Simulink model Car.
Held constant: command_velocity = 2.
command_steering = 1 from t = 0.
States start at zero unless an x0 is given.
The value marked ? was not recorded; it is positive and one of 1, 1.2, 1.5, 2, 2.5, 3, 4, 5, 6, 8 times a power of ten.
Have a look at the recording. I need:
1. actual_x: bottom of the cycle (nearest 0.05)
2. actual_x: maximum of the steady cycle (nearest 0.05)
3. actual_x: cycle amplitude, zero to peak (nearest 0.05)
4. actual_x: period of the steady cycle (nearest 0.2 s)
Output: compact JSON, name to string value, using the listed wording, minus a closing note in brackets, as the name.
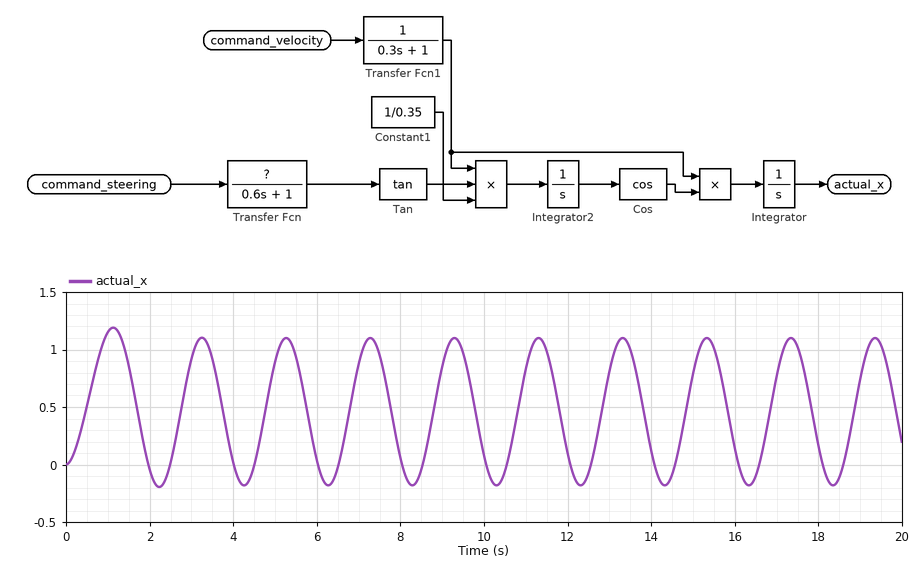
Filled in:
{"actual_x: bottom of the cycle": "-0.20", "actual_x: maximum of the steady cycle": "1.10", "actual_x: cycle amplitude, zero to peak": "0.65", "actual_x: period of the steady cycle": "2.0 s"}
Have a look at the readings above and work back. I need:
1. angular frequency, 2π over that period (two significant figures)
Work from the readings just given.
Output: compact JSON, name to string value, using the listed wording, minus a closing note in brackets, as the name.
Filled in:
{"angular frequency, 2π over that period": "3.1 rad/s"}
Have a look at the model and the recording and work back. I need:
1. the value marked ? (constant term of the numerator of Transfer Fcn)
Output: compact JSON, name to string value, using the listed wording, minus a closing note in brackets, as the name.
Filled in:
{"the value marked ?": "0.5"}
